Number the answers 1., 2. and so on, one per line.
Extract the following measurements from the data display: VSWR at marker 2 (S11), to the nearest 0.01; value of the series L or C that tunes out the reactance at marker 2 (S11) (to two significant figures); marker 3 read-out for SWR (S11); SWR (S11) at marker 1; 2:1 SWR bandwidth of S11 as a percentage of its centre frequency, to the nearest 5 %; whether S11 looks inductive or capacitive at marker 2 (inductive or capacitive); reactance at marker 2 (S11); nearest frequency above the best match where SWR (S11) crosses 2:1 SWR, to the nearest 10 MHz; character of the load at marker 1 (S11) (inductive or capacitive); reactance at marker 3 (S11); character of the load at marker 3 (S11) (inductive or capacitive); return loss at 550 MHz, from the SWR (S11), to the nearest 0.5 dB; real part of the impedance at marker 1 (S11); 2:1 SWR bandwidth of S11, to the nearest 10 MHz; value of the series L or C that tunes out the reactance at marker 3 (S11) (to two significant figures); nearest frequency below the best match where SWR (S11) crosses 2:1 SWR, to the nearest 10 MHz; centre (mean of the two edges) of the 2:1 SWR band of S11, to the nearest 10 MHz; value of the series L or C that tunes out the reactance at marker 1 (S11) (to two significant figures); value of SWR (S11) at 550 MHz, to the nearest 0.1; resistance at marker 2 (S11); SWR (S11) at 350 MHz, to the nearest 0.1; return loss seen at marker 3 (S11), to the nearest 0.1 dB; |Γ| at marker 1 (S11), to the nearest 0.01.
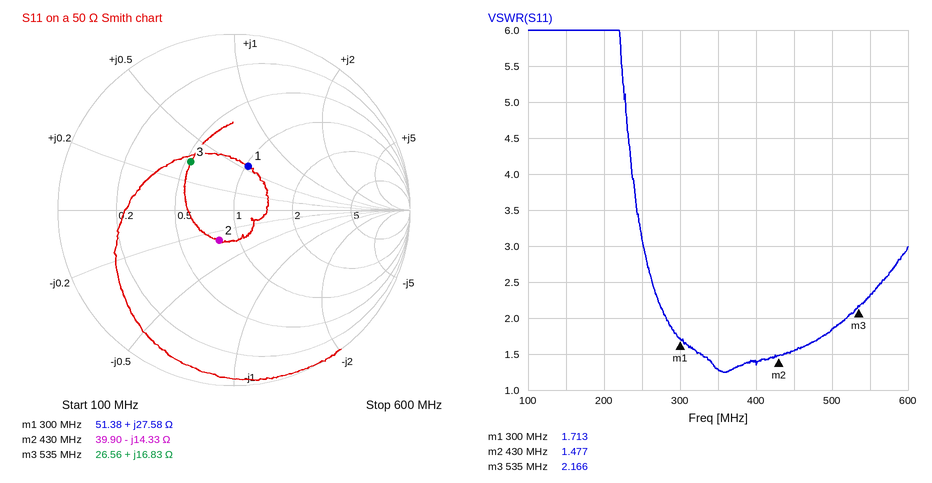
1. 1.48
2. 5.3 nH
3. 2.166
4. 1.713
5. 60 %
6. capacitive
7. -14.33 Ω
8. 520 MHz
9. inductive
10. +16.83 Ω
11. inductive
12. 8.0 dB
13. 51.38 Ω
14. 240 MHz
15. 18 pF
16. 280 MHz
17. 400 MHz
18. 19 pF
19. 2.3
20. 39.90 Ω
21. 1.3
22. 8.7 dB
23. 0.26
